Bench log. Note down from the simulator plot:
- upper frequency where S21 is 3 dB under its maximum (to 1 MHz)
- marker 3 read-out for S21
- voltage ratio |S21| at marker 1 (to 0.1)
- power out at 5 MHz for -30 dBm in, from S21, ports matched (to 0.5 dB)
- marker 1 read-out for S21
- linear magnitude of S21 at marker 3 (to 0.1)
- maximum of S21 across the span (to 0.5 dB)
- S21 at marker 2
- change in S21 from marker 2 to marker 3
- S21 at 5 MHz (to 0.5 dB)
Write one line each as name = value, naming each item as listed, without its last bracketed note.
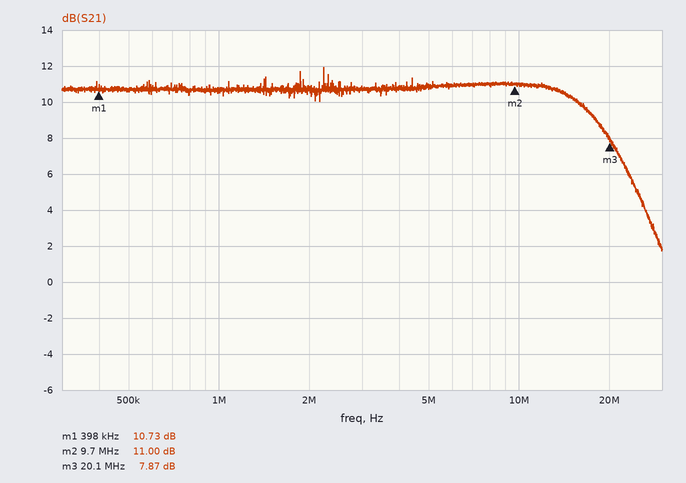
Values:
upper frequency where S21 is 3 dB under its maximum = 18 MHz
marker 3 read-out for S21 = 7.87 dB
voltage ratio |S21| at marker 1 = 3.4
power out at 5 MHz for -30 dBm in, from S21, ports matched = -19.0 dBm
marker 1 read-out for S21 = 10.73 dB
linear magnitude of S21 at marker 3 = 2.5
maximum of S21 across the span = 12.0 dB
S21 at marker 2 = 11.00 dB
change in S21 from marker 2 to marker 3 = -3.13 dB
S21 at 5 MHz = 11.0 dB
